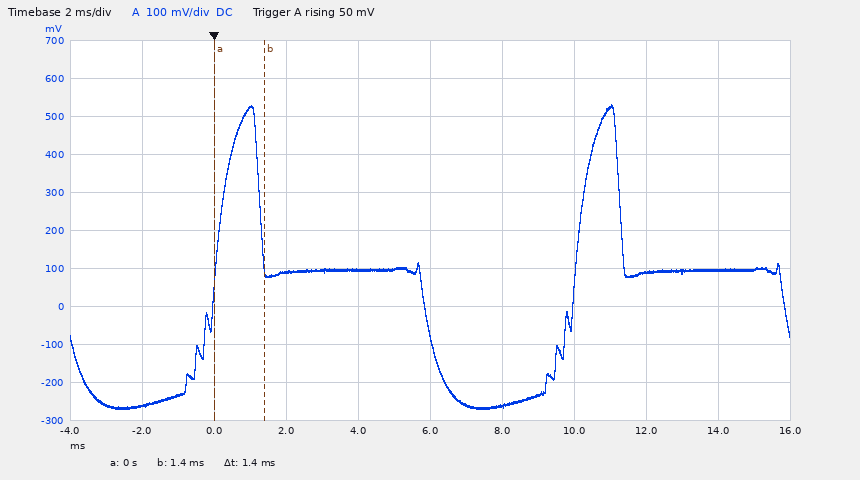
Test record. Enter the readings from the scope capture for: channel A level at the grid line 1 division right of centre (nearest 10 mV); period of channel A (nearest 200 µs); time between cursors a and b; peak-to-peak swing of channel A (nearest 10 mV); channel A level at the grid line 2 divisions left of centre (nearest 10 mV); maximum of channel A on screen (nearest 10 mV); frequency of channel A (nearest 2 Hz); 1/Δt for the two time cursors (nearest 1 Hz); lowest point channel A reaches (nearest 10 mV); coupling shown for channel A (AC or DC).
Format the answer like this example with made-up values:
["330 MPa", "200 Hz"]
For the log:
["-260 mV", "10.0 ms", "1.4 ms", "800 mV", "90 mV", "530 mV", "100 Hz", "714 Hz", "-270 mV", "DC"]
